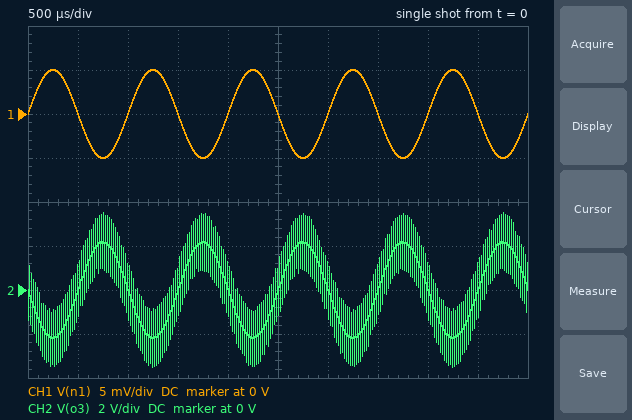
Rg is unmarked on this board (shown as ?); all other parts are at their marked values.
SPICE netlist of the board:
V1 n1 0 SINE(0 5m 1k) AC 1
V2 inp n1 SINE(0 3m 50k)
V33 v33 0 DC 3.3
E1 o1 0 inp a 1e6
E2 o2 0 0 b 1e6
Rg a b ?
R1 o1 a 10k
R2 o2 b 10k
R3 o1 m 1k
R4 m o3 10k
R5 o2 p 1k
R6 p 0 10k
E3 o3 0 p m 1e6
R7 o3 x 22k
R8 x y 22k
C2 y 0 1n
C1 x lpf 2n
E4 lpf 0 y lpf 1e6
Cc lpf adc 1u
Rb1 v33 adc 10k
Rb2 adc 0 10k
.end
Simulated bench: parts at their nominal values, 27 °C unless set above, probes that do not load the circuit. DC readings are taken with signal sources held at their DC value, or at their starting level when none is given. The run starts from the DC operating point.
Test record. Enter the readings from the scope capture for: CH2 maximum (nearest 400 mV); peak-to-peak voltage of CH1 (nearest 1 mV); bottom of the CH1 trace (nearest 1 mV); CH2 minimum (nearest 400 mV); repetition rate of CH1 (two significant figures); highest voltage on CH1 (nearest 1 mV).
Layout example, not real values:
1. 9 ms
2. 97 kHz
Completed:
1. 3.6 V
2. 10 mV
3. -5 mV
4. -3.6 V
5. 1.0 kHz
6. 5 mV
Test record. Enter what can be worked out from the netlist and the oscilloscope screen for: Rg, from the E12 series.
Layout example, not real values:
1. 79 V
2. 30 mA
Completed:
1. 470 Ω
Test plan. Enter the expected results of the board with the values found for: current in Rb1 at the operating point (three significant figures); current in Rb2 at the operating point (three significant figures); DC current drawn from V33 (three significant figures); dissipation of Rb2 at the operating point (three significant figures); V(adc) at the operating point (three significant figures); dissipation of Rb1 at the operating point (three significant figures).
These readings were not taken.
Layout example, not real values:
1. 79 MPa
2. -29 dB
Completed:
1. 165 µA
2. 165 µA
3. 165 µA
4. 272 µW
5. 1.65 V
6. 272 µW
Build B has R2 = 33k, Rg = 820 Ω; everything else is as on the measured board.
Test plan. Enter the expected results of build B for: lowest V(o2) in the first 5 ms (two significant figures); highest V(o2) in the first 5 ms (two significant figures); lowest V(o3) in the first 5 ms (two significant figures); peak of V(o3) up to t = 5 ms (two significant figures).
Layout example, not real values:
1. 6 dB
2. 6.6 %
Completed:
1. -320 mV
2. 320 mV
3. -4.3 V
4. 4.3 V
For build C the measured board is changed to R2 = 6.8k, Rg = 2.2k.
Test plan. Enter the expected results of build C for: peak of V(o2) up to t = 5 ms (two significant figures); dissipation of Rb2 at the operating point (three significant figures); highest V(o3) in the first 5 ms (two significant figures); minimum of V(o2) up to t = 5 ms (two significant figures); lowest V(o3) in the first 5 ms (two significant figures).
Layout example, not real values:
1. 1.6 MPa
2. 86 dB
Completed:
1. 25 mV
2. 272 µW
3. 690 mV
4. -25 mV
5. -690 mV
